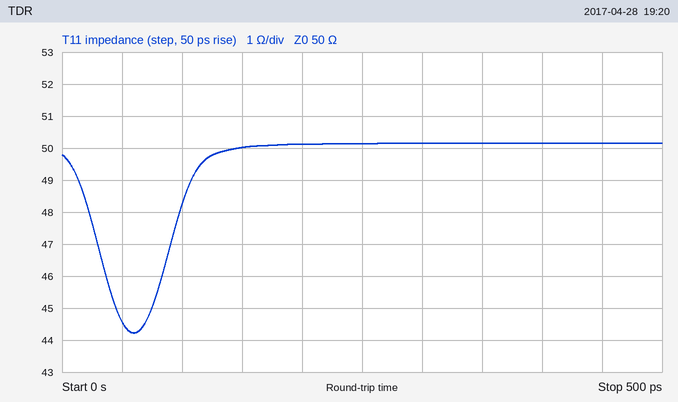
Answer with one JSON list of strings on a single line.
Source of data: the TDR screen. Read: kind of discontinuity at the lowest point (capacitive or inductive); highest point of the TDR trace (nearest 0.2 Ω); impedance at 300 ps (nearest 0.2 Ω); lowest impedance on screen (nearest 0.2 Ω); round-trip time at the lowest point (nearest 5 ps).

["capacitive", "50.2 Ω", "50.2 Ω", "44.2 Ω", "60 ps"]
